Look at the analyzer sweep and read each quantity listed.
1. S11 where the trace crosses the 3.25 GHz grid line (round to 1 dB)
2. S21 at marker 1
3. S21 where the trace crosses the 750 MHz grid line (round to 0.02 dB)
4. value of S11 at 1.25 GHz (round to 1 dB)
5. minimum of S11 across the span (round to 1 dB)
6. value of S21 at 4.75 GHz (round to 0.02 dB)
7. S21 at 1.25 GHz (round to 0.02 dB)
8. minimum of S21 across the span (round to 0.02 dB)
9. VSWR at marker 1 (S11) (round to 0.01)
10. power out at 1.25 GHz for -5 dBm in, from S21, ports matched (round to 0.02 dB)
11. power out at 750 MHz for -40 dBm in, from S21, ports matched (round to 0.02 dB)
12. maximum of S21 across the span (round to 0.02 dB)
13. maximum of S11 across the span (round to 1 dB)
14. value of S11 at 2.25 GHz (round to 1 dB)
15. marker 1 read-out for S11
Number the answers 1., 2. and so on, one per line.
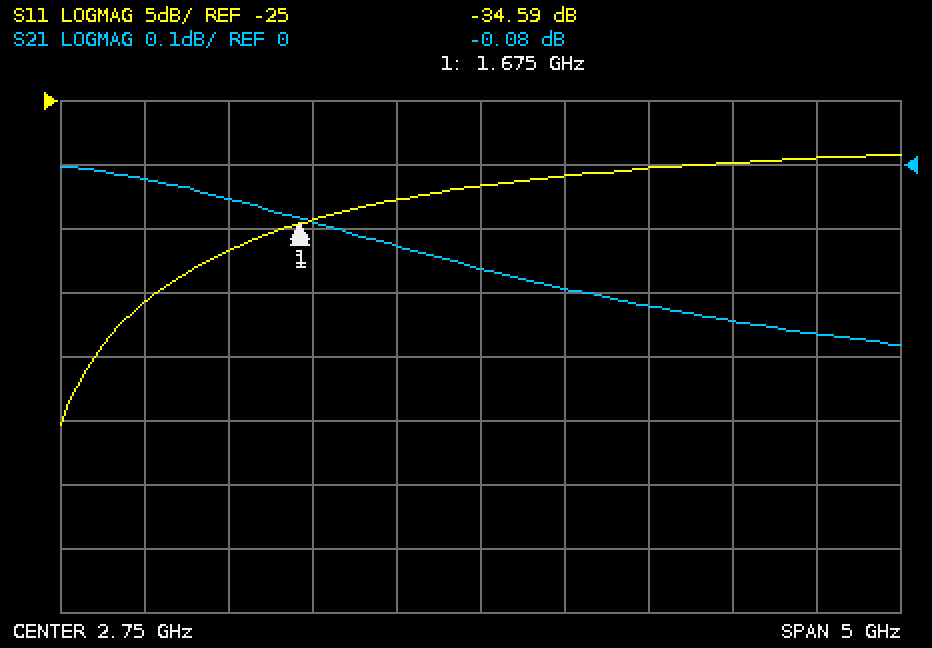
1. -31 dB
2. -0.08 dB
3. -0.02 dB
4. -37 dB
5. -50 dB
6. -0.26 dB
7. -0.06 dB
8. -0.28 dB
9. 1.04
10. -5.06 dBm
11. -40.02 dBm
12. 0.00 dB
13. -29 dB
14. -33 dB
15. -34.59 dB
